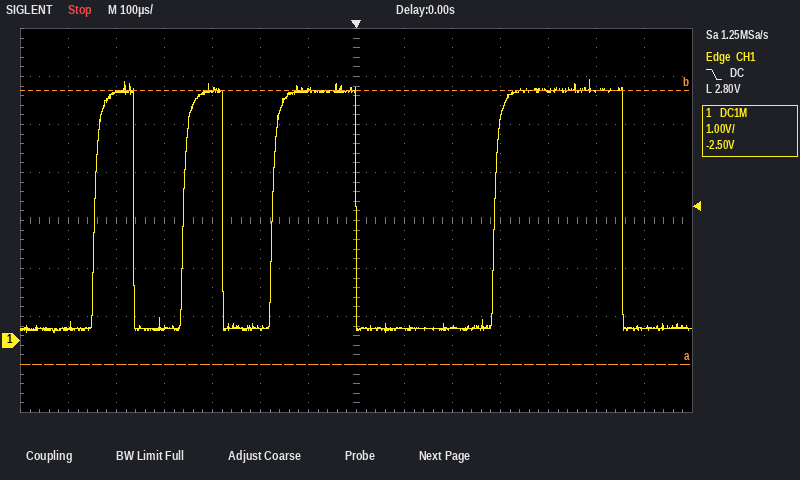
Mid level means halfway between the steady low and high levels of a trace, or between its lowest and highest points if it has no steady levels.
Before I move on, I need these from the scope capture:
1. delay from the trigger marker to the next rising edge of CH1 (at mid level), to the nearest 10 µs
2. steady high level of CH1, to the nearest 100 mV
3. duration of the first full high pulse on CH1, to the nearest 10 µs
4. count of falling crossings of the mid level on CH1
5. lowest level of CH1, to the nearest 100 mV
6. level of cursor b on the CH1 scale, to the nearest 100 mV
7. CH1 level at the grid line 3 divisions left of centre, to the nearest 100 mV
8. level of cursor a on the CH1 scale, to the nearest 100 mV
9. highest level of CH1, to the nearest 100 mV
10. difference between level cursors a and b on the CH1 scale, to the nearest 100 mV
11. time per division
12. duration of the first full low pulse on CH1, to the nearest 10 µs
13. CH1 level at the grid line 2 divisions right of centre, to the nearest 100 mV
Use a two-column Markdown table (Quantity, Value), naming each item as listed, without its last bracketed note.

| Quantity | Value |
|---|---|
| delay from the trigger marker to the next rising edge of CH1 (at mid level), to the nearest 10 µs | 290 µs |
| steady high level of CH1, to the nearest 100 mV | 5.2 V |
| duration of the first full high pulse on CH1, to the nearest 10 µs | 80 µs |
| count of falling crossings of the mid level on CH1 | 4 |
| lowest level of CH1, to the nearest 100 mV | 200 mV |
| level of cursor b on the CH1 scale, to the nearest 100 mV | 5.2 V |
| CH1 level at the grid line 3 divisions left of centre, to the nearest 100 mV | 5.2 V |
| level of cursor a on the CH1 scale, to the nearest 100 mV | -500 mV |
| highest level of CH1, to the nearest 100 mV | 5.4 V |
| difference between level cursors a and b on the CH1 scale, to the nearest 100 mV | 5.7 V |
| time per division | 100 µs |
| duration of the first full low pulse on CH1, to the nearest 10 µs | 100 µs |
| CH1 level at the grid line 2 divisions right of centre, to the nearest 100 mV | 300 mV |
